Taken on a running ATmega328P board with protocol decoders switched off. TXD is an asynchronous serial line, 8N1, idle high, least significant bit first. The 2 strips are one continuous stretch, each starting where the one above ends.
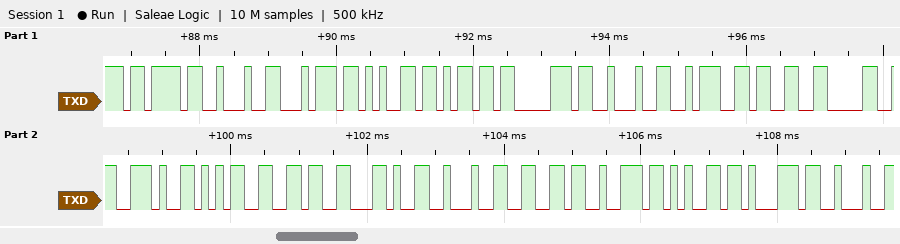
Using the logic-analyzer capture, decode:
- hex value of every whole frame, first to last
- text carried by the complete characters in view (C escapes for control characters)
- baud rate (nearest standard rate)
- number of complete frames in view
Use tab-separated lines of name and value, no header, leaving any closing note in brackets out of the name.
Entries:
hex value of every whole frame, first to last	0x7B 0x22 0x74 0x65 0x6D 0x70 0x22 0x3A 0x33 0x30 0x2E 0x35 0x36 0x2C 0x22 0x66 0x72 0x65 0x71 0x22
text carried by the complete characters in view	"{\"temp\":30.56,\"freq\""
baud rate	9600 baud
number of complete frames in view	20
